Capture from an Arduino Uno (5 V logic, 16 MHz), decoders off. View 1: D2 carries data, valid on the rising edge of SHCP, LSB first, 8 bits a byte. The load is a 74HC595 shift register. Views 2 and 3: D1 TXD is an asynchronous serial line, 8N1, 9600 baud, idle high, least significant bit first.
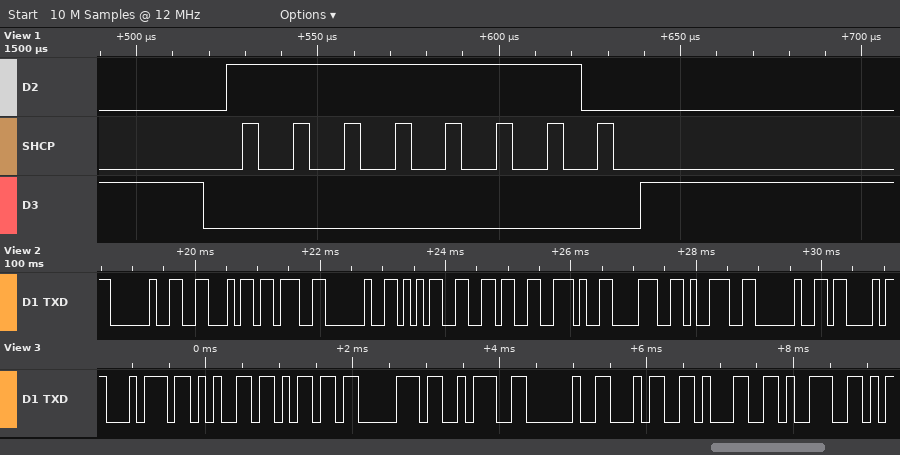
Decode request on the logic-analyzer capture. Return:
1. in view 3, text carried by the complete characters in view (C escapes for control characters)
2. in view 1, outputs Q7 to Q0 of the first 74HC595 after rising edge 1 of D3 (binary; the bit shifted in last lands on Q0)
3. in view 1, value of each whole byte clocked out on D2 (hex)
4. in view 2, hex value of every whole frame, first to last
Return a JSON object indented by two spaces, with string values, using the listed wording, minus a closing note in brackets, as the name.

{
  "in view 3, text carried by the complete characters in view": "\"temp: 419\"",
  "in view 1, outputs Q7 to Q0 of the first 74HC595 after rising edge 1 of D3": "11111110",
  "in view 1, value of each whole byte clocked out on D2": "0x7F",
  "in view 2, hex value of every whole frame, first to last": "20 46 3B 20 35 36 2E 38 39 20 43"
}
